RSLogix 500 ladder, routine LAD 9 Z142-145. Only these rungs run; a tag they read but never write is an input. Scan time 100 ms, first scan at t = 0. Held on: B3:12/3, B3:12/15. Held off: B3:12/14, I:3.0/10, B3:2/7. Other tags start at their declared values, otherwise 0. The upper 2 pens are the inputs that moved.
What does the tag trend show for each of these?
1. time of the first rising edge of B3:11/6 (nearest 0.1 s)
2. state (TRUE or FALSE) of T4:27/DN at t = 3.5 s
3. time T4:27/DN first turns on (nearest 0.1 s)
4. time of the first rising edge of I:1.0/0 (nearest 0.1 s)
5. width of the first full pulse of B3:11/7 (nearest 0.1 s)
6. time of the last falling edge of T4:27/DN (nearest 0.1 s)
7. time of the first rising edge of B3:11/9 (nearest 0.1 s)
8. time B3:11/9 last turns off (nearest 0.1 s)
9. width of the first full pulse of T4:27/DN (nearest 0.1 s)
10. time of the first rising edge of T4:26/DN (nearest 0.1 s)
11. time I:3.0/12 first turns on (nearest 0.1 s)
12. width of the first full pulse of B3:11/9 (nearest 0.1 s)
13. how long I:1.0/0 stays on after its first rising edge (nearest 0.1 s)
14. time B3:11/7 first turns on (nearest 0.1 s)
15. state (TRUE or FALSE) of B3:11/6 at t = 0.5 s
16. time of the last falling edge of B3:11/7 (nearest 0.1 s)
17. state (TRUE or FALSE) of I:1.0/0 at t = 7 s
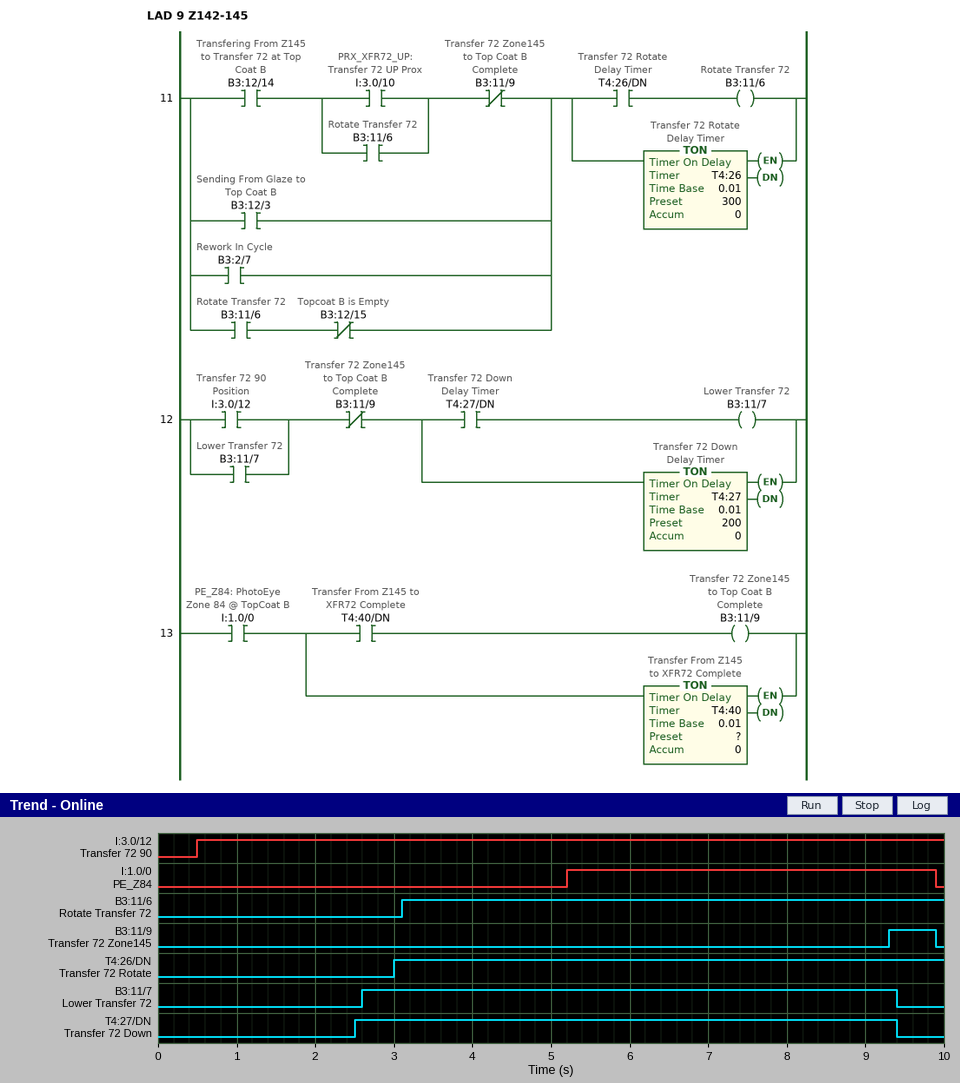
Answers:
3.1 s
TRUE
2.5 s
5.2 s
6.8 s
9.4 s
9.3 s
9.9 s
6.9 s
3.0 s
0.5 s
0.6 s
4.7 s
2.6 s
FALSE
9.4 s
TRUE
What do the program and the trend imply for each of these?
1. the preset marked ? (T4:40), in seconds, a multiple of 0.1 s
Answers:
4.0 s
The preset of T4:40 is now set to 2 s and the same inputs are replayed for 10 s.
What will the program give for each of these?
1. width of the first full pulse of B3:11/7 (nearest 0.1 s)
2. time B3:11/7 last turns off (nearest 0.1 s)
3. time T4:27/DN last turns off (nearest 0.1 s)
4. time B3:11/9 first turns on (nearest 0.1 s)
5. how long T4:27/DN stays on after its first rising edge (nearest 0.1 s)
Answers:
4.8 s
7.4 s
7.4 s
7.3 s
4.9 s
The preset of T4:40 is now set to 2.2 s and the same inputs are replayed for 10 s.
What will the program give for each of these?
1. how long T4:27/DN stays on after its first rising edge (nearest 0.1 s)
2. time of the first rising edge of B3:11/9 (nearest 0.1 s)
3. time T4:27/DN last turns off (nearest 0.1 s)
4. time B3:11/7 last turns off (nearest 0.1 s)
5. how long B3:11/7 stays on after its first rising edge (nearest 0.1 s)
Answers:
5.1 s
7.5 s
7.6 s
7.6 s
5.0 s
